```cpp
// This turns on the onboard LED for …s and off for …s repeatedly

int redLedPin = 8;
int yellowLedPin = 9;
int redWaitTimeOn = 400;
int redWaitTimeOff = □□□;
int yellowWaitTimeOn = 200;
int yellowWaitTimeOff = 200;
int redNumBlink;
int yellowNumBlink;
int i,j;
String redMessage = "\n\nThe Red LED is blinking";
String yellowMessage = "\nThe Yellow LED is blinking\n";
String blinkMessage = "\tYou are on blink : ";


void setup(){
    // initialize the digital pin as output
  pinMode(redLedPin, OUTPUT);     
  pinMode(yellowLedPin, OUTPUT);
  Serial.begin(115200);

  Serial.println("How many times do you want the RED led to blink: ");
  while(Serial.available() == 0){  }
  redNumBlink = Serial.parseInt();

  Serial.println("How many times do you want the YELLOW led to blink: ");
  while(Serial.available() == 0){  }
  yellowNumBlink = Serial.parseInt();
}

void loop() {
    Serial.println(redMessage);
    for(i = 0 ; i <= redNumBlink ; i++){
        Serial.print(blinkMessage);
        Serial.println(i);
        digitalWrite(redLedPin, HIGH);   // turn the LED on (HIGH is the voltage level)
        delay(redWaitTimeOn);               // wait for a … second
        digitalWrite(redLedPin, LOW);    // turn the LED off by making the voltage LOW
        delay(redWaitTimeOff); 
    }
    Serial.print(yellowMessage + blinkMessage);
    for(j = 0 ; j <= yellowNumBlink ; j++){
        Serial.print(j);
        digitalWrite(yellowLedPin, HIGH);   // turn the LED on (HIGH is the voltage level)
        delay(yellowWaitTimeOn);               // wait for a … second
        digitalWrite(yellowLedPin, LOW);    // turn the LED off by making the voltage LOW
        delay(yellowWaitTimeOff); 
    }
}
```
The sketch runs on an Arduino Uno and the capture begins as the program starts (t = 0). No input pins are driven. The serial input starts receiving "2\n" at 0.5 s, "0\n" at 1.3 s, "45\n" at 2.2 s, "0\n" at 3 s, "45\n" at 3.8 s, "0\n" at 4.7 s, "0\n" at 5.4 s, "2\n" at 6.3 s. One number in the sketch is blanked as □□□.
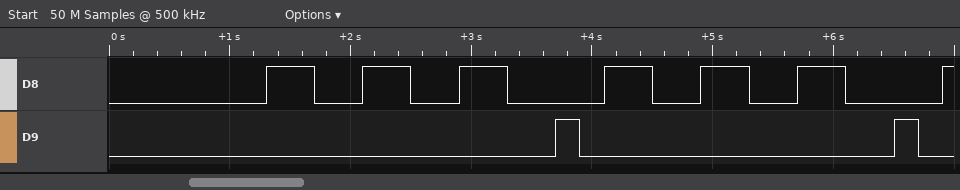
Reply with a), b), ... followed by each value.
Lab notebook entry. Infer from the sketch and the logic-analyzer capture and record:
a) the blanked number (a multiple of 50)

a) 400
